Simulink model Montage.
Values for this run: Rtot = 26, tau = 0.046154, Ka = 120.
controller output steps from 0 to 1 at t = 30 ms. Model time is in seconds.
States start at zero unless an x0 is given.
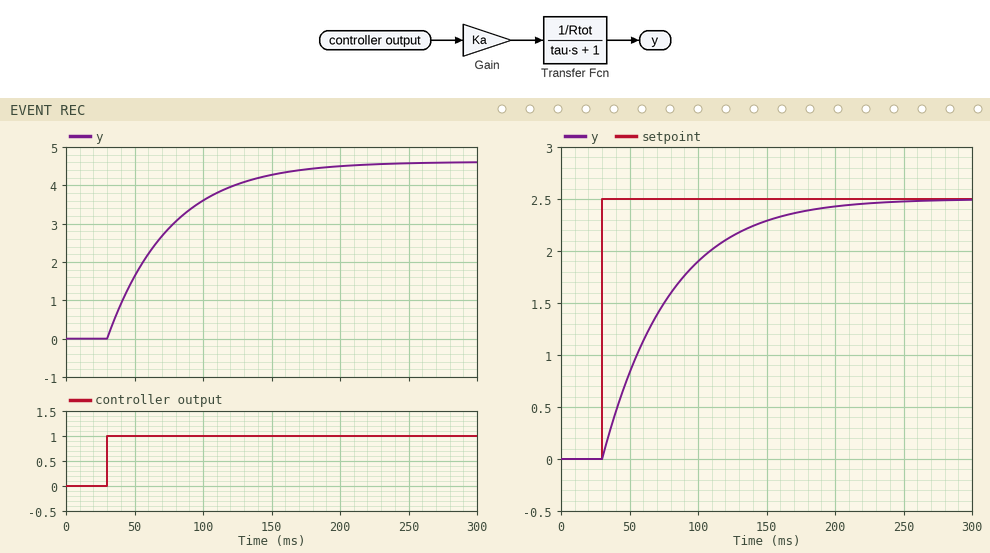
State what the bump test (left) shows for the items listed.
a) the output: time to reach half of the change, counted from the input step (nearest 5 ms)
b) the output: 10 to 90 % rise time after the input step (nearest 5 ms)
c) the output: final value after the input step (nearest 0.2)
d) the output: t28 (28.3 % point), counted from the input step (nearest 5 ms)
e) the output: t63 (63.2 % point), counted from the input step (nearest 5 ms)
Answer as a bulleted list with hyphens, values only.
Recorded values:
- 30 ms
- 100 ms
- 4.6
- 15 ms
- 45 ms
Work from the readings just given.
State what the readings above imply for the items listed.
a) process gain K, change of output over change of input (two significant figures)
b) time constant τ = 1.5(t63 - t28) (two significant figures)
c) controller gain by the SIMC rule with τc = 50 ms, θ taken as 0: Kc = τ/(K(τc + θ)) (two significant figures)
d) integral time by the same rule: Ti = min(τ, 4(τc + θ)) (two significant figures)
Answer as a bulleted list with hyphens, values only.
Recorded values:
- 4.6
- 45 ms
- 0.20
- 45 ms
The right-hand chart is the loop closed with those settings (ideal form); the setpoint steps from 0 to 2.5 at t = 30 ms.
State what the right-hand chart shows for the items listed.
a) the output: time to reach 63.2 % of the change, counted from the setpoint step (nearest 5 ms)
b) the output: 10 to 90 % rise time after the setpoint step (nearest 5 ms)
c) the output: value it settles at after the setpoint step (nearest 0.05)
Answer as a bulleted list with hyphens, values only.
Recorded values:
- 50 ms
- 105 ms
- 2.50
